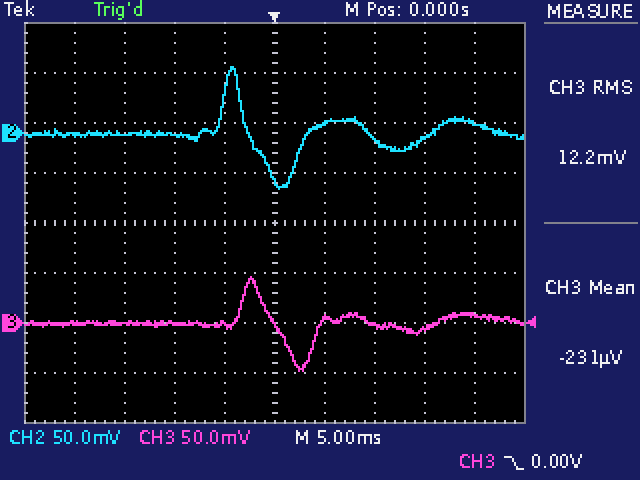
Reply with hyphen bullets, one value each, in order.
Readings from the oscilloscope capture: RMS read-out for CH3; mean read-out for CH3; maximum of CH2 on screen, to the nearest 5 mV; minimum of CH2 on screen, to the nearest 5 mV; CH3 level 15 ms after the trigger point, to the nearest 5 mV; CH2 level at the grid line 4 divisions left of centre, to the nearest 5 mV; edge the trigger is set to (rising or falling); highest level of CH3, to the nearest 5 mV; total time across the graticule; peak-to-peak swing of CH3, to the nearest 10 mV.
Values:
- 12.2 mV
- -231 µV
- 65 mV
- -55 mV
- -5 mV
- 0 mV
- falling
- 45 mV
- 50 ms
- 90 mV
